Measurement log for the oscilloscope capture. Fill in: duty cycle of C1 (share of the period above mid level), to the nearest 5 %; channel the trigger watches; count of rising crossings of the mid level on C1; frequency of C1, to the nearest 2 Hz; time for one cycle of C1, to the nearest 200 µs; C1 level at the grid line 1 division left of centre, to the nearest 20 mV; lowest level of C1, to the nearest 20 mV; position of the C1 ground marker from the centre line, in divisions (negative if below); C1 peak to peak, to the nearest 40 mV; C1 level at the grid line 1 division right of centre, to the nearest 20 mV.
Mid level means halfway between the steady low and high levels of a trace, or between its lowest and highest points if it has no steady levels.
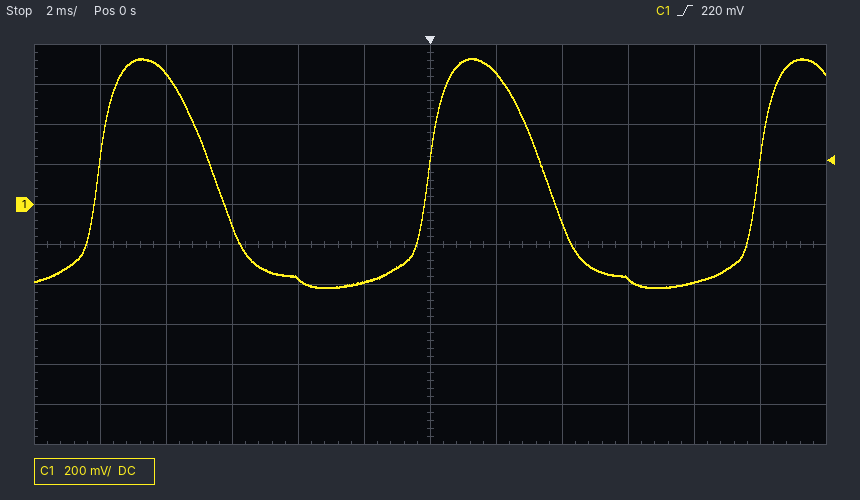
35 %
C1
3
100 Hz
10.0 ms
-380 mV
-420 mV
+1.0 div
1.16 V
660 mV
